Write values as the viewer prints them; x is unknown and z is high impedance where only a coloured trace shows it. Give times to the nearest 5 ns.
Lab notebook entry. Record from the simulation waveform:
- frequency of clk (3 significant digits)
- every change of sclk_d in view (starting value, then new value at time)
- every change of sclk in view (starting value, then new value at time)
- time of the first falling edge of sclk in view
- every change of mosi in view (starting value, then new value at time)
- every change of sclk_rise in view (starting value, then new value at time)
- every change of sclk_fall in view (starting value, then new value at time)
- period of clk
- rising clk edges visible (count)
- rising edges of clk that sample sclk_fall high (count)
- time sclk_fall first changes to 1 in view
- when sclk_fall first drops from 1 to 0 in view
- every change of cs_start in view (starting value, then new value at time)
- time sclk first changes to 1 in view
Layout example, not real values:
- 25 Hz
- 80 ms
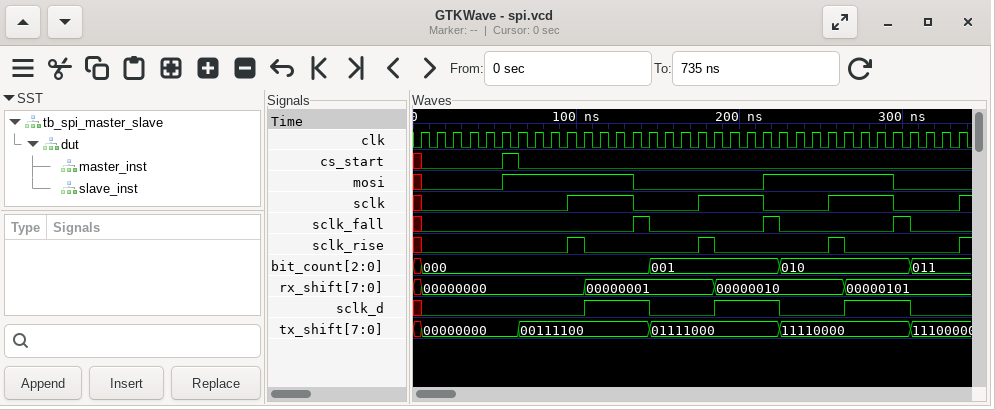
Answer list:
- 100 MHz
- x, 0 at 5 ns, 1 at 105 ns, 0 at 145 ns, 1 at 185 ns, 0 at 225 ns, 1 at 265 ns, 0 at 305 ns
- x, 0 at 5 ns, 1 at 95 ns, 0 at 135 ns, 1 at 175 ns, 0 at 215 ns, 1 at 255 ns, 0 at 295 ns, 1 at 335 ns
- 135 ns
- x, 0 at 5 ns, 1 at 55 ns, 0 at 135 ns, 1 at 215 ns, 0 at 295 ns
- x, 0 at 5 ns, 1 at 95 ns, 0 at 105 ns, 1 at 175 ns, 0 at 185 ns, 1 at 255 ns, 0 at 265 ns, 1 at 335 ns
- x, 0 at 5 ns, 1 at 135 ns, 0 at 145 ns, 1 at 215 ns, 0 at 225 ns, 1 at 295 ns, 0 at 305 ns
- 10 ns
- 34
- 3
- 135 ns
- 145 ns
- x, 0 at 5 ns, 1 at 55 ns, 0 at 65 ns
- 95 ns
